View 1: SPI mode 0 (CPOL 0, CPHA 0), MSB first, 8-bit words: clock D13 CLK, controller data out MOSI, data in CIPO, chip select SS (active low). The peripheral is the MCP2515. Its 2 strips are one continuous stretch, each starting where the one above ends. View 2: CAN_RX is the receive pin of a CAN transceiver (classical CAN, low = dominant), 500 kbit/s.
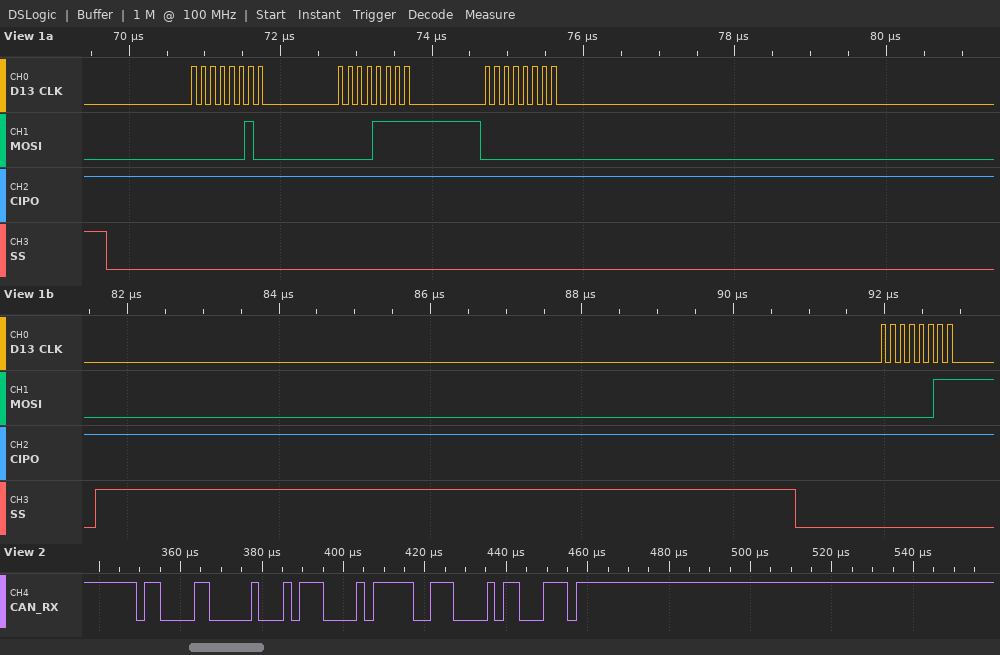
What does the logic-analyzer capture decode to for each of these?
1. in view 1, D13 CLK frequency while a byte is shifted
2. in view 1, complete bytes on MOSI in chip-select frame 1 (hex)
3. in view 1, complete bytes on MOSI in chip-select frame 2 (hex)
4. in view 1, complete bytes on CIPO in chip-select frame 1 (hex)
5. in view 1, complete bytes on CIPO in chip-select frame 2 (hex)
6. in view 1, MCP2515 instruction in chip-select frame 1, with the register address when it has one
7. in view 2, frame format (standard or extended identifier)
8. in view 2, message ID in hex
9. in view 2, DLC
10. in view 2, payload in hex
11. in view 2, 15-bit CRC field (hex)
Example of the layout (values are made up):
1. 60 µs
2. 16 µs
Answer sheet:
1. 8 MHz
2. 0x02 0x0F 0x00
3. 0x03
4. 0xFF 0xFF 0xFF
5. 0xFF
6. WRITE 0x0F
7. standard
8. 0x618
9. 2
10. E1 7D
11. 0x6163
